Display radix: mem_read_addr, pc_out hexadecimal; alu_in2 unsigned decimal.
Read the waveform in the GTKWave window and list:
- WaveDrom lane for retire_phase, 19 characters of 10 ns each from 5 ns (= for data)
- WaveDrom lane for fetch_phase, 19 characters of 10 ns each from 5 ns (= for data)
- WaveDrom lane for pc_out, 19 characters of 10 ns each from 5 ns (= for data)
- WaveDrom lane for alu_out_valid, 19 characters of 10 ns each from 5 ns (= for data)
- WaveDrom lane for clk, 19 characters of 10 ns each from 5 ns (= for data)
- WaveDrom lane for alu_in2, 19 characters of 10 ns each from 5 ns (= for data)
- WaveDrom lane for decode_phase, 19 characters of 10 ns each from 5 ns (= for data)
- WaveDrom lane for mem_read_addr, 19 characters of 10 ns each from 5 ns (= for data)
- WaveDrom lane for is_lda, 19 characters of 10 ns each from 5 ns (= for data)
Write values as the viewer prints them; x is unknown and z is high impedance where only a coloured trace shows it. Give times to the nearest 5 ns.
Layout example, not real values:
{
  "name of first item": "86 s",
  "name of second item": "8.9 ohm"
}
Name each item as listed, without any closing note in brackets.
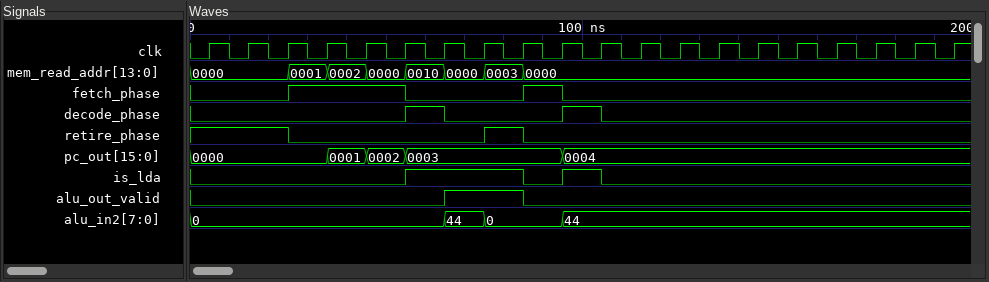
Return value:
{
  "WaveDrom lane for retire_phase, 19 characters of 10 ns each from 5 ns": "{name: 'retire_phase', wave: '1.0....10..........'}",
  "WaveDrom lane for fetch_phase, 19 characters of 10 ns each from 5 ns": "{name: 'fetch_phase', wave: '0.1..0..10.........'}",
  "WaveDrom lane for pc_out, 19 characters of 10 ns each from 5 ns": "{name: 'pc_out', wave: '=..===...=.........', data: '0000 0001 0002 0003 0004'}",
  "WaveDrom lane for alu_out_valid, 19 characters of 10 ns each from 5 ns": "{name: 'alu_out_valid', wave: '0.....1.0..........'}",
  "WaveDrom lane for clk, 19 characters of 10 ns each from 5 ns": "{name: 'clk', wave: 'p..................'}",
  "WaveDrom lane for alu_in2, 19 characters of 10 ns each from 5 ns": "{name: 'alu_in2', wave: '=.....==.=.........', data: '0 44 0 44'}",
  "WaveDrom lane for decode_phase, 19 characters of 10 ns each from 5 ns": "{name: 'decode_phase', wave: '0....10..10........'}",
  "WaveDrom lane for mem_read_addr, 19 characters of 10 ns each from 5 ns": "{name: 'mem_read_addr', wave: '=.=======..........', data: '0000 0001 0002 0000 0010 0000 0003 0000'}",
  "WaveDrom lane for is_lda, 19 characters of 10 ns each from 5 ns": "{name: 'is_lda', wave: '0....1..010........'}"
}
